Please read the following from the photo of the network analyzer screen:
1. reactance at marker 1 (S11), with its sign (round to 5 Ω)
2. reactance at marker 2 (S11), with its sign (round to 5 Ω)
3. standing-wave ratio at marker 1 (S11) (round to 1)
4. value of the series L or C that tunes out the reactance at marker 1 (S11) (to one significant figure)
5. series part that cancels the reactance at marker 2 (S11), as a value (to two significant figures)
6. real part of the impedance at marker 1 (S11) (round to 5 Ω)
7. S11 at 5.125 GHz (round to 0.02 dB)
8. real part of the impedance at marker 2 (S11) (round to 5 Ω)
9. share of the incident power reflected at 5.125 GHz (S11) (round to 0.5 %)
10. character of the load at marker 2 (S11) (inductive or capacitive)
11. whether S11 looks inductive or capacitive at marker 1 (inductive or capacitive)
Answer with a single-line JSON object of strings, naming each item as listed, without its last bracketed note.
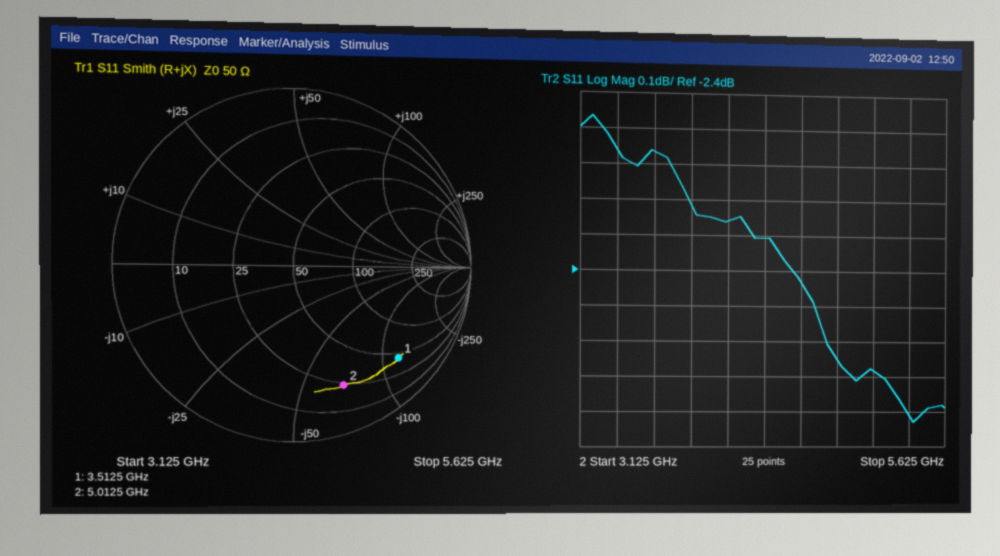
{"reactance at marker 1 (S11), with its sign": "-120 Ω", "reactance at marker 2 (S11), with its sign": "-70 Ω", "standing-wave ratio at marker 1 (S11)": "8", "value of the series L or C that tunes out the reactance at marker 1 (S11)": "5 nH", "series part that cancels the reactance at marker 2 (S11), as a value": "2.2 nH", "real part of the impedance at marker 1 (S11)": "45 Ω", "S11 at 5.125 GHz": "-2.68 dB", "real part of the impedance at marker 2 (S11)": "25 Ω", "share of the incident power reflected at 5.125 GHz (S11)": "54.0 %", "character of the load at marker 2 (S11)": "capacitive", "whether S11 looks inductive or capacitive at marker 1": "capacitive"}
